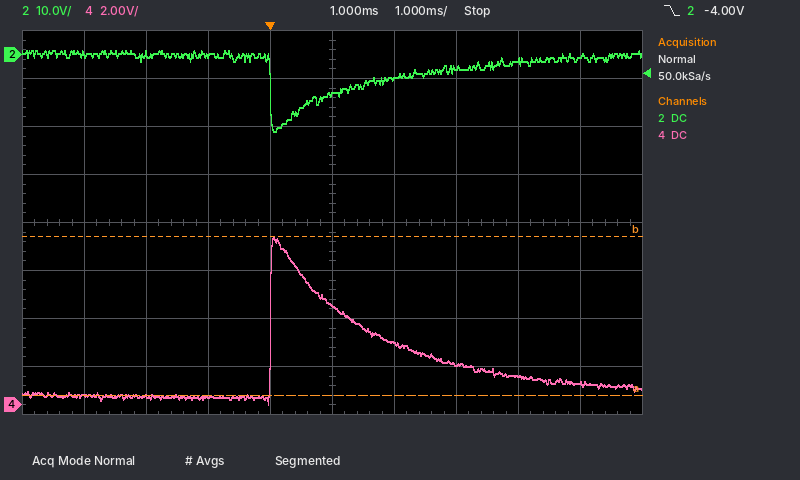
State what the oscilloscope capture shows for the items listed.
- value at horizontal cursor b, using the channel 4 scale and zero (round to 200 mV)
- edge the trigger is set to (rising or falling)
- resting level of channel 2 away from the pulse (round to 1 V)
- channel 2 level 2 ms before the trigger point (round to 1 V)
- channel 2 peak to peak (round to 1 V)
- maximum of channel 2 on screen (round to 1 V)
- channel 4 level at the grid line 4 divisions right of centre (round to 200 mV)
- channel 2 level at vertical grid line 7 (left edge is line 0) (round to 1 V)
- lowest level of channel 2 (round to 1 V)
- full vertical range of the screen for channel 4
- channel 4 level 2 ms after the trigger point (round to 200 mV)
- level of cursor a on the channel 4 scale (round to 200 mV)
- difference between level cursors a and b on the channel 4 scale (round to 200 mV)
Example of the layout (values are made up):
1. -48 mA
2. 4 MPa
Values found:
1. 7.0 V
2. falling
3. 0 V
4. 0 V
5. 17 V
6. 1 V
7. 800 mV
8. -3 V
9. -16 V
10. 16 V
11. 2.6 V
12. 400 mV
13. 6.6 V
